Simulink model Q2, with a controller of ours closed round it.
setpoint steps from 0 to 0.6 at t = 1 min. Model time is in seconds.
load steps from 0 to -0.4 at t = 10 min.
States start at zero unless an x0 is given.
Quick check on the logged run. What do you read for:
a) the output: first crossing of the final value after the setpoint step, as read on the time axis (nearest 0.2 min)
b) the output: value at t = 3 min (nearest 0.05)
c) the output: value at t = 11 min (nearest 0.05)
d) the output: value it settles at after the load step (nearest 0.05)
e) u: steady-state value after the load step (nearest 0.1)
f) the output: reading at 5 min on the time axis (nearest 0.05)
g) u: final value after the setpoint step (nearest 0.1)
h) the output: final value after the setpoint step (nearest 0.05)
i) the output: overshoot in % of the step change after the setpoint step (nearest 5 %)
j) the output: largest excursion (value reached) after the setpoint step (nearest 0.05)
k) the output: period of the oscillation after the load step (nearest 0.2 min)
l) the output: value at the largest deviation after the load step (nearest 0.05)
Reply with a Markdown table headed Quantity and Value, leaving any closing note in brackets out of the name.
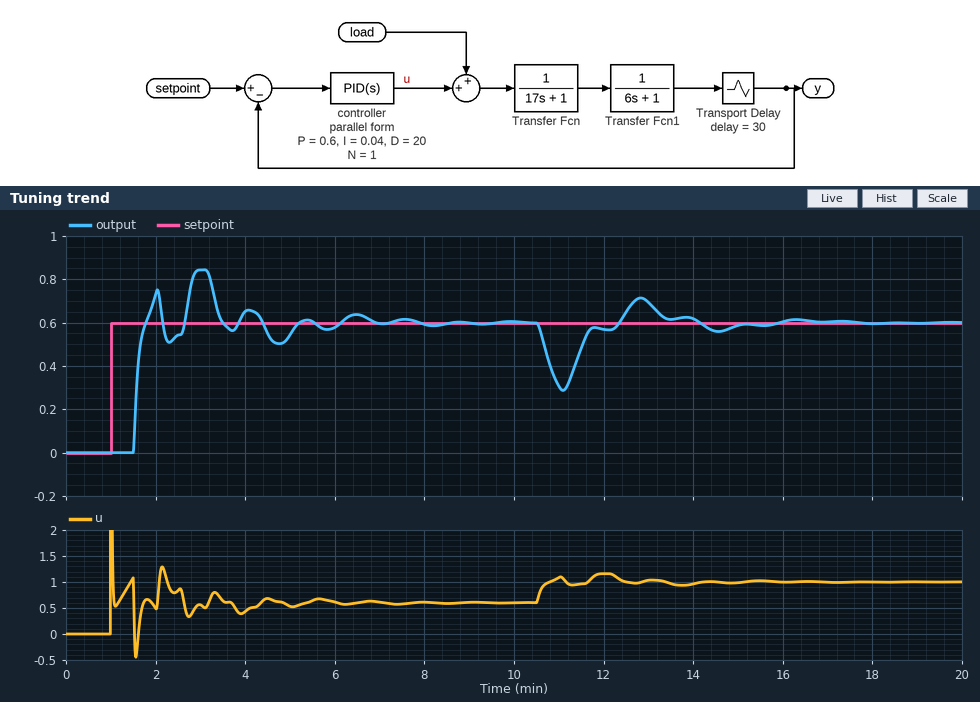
| Quantity | Value |
|---|---|
| the output: first crossing of the final value after the setpoint step, as read on the time axis | 1.8 min |
| the output: value at t = 3 min | 0.85 |
| the output: value at t = 11 min | 0.30 |
| the output: value it settles at after the load step | 0.60 |
| u: steady-state value after the load step | 1.0 |
| the output: reading at 5 min on the time axis | 0.55 |
| u: final value after the setpoint step | 0.6 |
| the output: final value after the setpoint step | 0.60 |
| the output: overshoot in % of the step change after the setpoint step | 40 % |
| the output: largest excursion (value reached) after the setpoint step | 0.85 |
| the output: period of the oscillation after the load step | 3.4 min |
| the output: value at the largest deviation after the load step | 0.30 |
